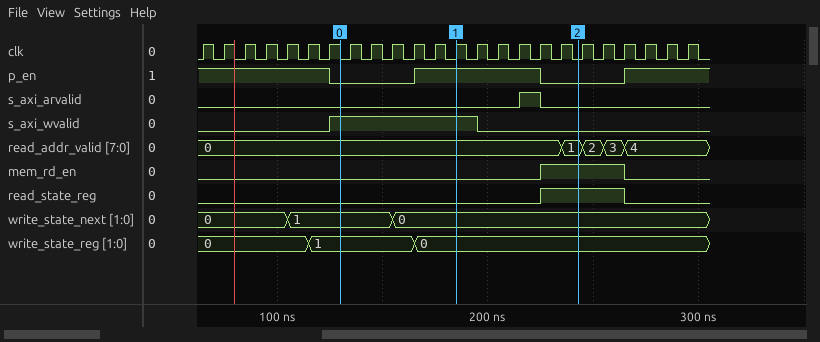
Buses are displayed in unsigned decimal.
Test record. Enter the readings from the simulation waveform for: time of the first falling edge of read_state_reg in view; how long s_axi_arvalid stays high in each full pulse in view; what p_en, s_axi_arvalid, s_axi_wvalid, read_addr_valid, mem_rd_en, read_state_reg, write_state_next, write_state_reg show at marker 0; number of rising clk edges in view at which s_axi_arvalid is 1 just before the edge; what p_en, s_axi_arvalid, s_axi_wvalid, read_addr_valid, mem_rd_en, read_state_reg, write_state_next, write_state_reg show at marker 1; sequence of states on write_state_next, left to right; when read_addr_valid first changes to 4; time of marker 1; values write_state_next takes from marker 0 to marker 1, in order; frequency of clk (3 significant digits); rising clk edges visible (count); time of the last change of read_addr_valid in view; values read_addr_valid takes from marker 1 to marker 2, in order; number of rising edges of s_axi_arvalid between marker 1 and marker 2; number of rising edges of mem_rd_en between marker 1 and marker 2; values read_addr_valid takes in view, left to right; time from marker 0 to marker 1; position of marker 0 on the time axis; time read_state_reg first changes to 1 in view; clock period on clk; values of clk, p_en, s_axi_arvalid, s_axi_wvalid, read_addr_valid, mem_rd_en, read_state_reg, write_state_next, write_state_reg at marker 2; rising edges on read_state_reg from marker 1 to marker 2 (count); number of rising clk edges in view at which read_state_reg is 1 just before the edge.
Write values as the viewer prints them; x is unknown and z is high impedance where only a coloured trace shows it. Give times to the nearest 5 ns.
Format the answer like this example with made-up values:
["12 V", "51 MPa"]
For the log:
["265 ns", "10 ns", "p_en=0, s_axi_arvalid=0, s_axi_wvalid=1, read_addr_valid=0, mem_rd_en=0, read_state_reg=0, write_state_next=1, write_state_reg=1", "1", "p_en=1, s_axi_arvalid=0, s_axi_wvalid=1, read_addr_valid=0, mem_rd_en=0, read_state_reg=0, write_state_next=0, write_state_reg=0", "0, 1, 0", "265 ns", "185 ns", "1, 0", "100 MHz", "24", "265 ns", "0, 1", "1", "1", "0, 1, 2, 3, 4", "55 ns", "130 ns", "225 ns", "10 ns", "clk=0, p_en=0, s_axi_arvalid=0, s_axi_wvalid=0, read_addr_valid=1, mem_rd_en=1, read_state_reg=1, write_state_next=0, write_state_reg=0", "1", "4"]
